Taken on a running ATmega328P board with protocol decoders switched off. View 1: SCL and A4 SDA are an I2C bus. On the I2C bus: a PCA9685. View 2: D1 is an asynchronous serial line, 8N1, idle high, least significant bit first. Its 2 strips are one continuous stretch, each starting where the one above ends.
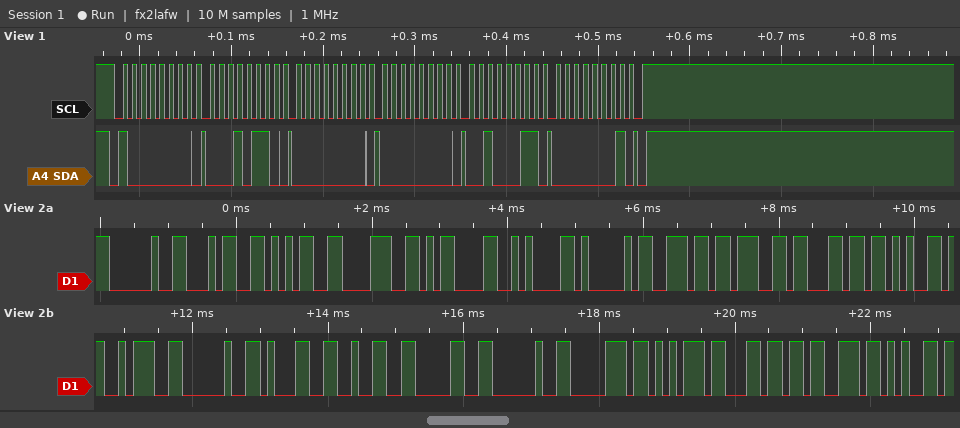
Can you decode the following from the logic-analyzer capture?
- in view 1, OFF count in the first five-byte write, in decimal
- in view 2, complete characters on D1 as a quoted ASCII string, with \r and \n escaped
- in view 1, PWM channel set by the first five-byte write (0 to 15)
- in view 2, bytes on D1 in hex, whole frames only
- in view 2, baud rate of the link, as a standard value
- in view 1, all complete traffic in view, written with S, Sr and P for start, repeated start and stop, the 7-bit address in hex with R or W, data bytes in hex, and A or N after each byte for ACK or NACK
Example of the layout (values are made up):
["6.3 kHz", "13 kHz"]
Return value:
["291", "\" 458\\r\\nAngle: 120 pulse\"", "4", "20 34 35 38 0D 0A 41 6E 67 6C 65 3A 20 31 32 30 20 70 75 6C 73 65", "9600 baud", "S 40W A 16 A 00 A 00 A 23 A 01 A P"]
